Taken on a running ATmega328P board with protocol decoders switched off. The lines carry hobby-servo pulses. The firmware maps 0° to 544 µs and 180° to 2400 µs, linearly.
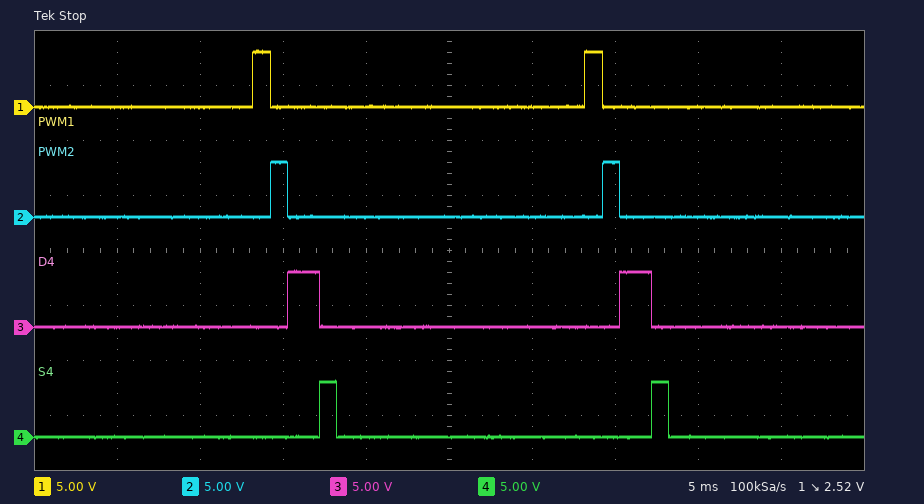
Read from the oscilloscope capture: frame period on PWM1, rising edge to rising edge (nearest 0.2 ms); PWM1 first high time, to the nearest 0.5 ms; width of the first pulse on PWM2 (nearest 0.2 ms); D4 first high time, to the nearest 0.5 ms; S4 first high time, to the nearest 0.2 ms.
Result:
20.0 ms
1.0 ms
1.0 ms
2.0 ms
1.0 ms
